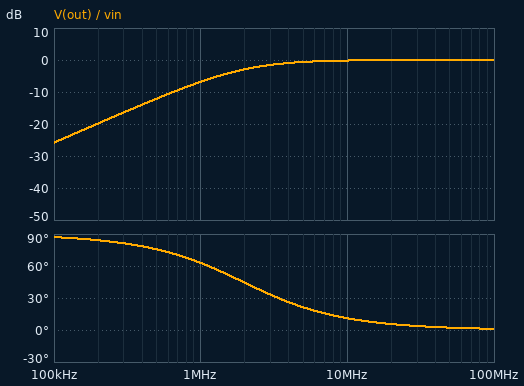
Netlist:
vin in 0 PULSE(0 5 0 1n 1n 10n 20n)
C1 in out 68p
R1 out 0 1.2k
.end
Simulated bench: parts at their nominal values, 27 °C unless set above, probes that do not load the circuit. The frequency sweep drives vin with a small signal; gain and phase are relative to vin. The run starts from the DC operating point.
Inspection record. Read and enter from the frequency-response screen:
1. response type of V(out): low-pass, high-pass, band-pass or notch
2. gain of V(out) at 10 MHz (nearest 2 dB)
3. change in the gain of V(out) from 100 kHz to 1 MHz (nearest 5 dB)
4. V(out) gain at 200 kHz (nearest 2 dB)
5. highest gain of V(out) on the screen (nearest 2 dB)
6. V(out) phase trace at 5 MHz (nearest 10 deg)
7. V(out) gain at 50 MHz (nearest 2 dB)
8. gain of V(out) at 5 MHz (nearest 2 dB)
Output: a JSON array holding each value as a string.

["high-pass", "0 dB", "20 dB", "-20 dB", "0 dB", "20 deg", "0 dB", "0 dB"]
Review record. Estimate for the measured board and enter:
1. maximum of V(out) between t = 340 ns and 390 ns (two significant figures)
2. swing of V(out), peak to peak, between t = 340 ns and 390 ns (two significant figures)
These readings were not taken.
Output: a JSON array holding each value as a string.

["2.4 V", "5.3 V"]
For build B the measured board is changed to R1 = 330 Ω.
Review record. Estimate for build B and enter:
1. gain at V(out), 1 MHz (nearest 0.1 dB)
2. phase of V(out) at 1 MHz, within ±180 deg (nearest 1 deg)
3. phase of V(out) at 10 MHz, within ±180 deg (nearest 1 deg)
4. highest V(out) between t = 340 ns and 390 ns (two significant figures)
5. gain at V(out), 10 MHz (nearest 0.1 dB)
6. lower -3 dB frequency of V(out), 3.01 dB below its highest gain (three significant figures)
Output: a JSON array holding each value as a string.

["-17.1 dB", "82 deg", "35 deg", "2.7 V", "-1.8 dB", "7.09 MHz"]
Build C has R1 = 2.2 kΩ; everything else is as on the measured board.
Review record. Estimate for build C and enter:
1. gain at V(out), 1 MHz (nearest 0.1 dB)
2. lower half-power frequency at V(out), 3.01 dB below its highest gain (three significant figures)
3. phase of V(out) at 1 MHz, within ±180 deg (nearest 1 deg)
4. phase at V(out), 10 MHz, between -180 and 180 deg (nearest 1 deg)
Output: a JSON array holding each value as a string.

["-3.3 dB", "1.06 MHz", "47 deg", "6 deg"]
